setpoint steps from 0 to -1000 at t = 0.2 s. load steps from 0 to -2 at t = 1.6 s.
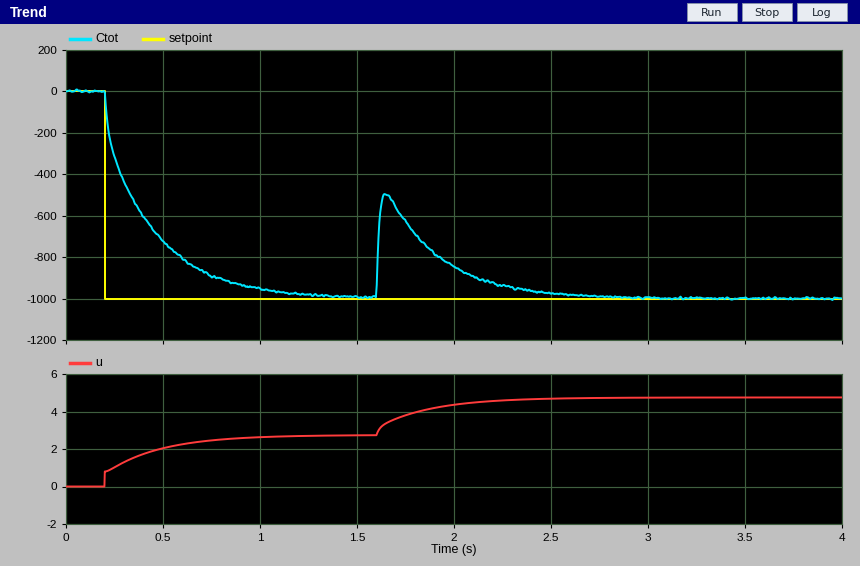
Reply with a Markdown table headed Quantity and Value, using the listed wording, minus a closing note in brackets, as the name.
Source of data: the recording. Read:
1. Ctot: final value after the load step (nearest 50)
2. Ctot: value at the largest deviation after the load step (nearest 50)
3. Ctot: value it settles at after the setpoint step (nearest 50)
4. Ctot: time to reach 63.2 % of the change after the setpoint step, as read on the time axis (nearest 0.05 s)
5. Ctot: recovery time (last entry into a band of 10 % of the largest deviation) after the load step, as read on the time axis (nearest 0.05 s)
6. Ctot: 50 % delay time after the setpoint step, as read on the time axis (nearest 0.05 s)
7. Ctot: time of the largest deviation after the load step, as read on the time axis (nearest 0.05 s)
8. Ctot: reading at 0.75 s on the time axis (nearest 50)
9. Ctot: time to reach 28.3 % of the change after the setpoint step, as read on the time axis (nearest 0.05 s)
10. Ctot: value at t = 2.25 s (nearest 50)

| Quantity | Value |
|---|---|
| Ctot: final value after the load step | -1000 |
| Ctot: value at the largest deviation after the load step | -500 |
| Ctot: value it settles at after the setpoint step | -1000 |
| Ctot: time to reach 63.2 % of the change after the setpoint step, as read on the time axis | 0.40 s |
| Ctot: recovery time (last entry into a band of 10 % of the largest deviation) after the load step, as read on the time axis | 2.30 s |
| Ctot: 50 % delay time after the setpoint step, as read on the time axis | 0.35 s |
| Ctot: time of the largest deviation after the load step, as read on the time axis | 1.65 s |
| Ctot: reading at 0.75 s on the time axis | -900 |
| Ctot: time to reach 28.3 % of the change after the setpoint step, as read on the time axis | 0.25 s |
| Ctot: value at t = 2.25 s | -950 |
